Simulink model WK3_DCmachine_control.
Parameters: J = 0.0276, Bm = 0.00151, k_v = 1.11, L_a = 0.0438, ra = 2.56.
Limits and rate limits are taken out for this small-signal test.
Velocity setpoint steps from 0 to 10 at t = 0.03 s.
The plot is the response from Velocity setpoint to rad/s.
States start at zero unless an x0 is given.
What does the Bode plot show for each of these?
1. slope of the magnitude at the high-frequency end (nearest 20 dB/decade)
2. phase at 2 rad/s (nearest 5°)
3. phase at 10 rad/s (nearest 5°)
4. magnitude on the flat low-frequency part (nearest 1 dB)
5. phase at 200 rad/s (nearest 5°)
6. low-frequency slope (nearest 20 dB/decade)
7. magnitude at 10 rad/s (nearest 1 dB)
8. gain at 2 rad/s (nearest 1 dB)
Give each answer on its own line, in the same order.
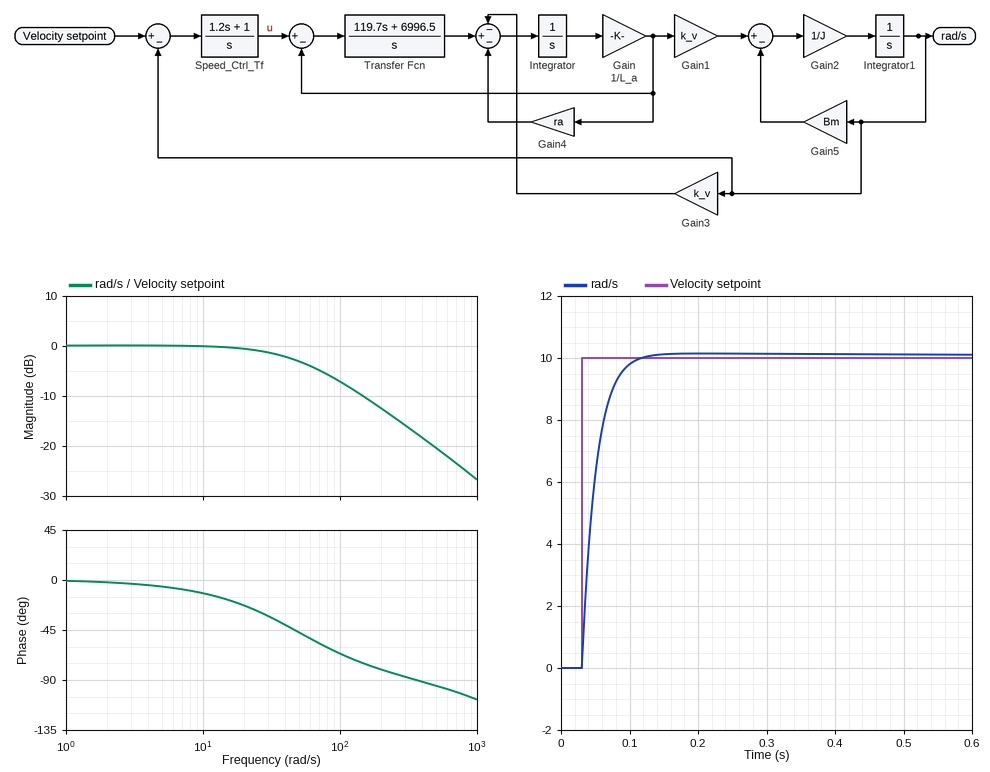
-20 dB/decade
0°
-10°
0 dB
-80°
0 dB/decade
0 dB
0 dB
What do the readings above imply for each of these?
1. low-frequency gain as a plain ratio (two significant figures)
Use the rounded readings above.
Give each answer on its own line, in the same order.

1.0
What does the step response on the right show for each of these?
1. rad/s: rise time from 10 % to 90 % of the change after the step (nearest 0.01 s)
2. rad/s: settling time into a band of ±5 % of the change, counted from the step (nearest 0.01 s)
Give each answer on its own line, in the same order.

0.04 s
0.06 s
